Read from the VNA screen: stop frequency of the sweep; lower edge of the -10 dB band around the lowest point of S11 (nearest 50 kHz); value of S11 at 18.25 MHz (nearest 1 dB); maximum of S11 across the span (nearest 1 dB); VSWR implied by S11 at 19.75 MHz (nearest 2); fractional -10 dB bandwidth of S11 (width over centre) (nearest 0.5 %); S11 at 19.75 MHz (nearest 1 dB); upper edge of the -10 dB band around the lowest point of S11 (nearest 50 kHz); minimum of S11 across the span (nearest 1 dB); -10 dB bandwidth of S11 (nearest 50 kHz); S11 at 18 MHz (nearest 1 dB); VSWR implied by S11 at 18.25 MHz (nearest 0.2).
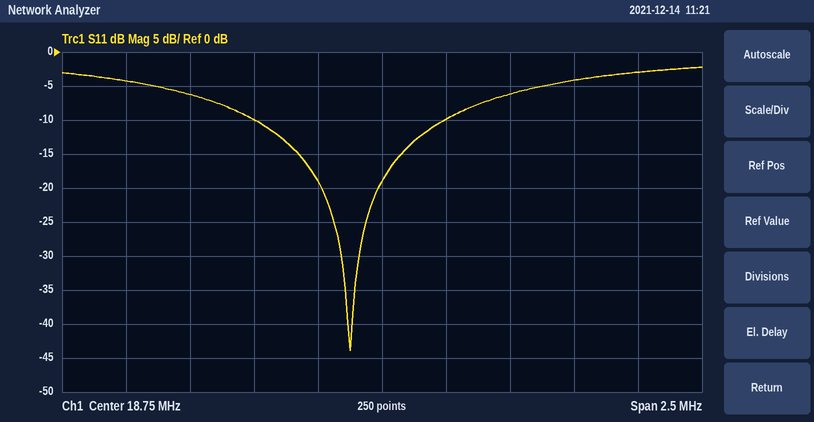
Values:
20 MHz
18.25 MHz
-10 dB
-2 dB
6
4.0 %
-3 dB
19.00 MHz
-44 dB
750 kHz
-6 dB
2.0
